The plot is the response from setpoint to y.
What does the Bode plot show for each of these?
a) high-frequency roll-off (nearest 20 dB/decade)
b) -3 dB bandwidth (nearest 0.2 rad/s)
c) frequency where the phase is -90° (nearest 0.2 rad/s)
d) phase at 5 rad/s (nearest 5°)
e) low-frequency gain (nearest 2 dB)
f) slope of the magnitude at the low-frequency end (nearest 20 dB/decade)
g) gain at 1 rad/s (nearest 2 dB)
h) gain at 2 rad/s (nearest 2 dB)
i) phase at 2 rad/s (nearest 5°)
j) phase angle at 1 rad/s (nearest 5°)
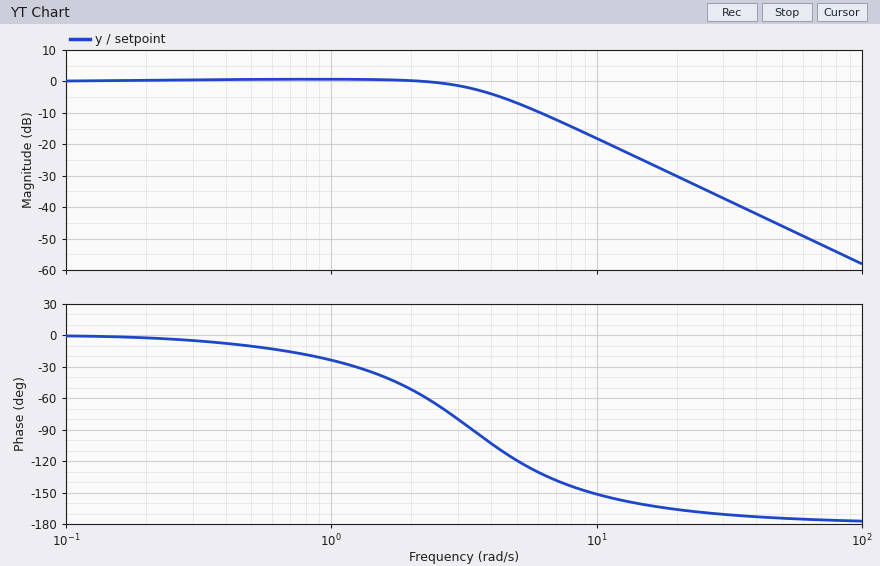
-40 dB/decade
3.6 rad/s
3.4 rad/s
-120°
0 dB
0 dB/decade
0 dB
0 dB
-50°
-25°
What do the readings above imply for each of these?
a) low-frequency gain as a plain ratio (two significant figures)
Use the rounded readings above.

1.0
